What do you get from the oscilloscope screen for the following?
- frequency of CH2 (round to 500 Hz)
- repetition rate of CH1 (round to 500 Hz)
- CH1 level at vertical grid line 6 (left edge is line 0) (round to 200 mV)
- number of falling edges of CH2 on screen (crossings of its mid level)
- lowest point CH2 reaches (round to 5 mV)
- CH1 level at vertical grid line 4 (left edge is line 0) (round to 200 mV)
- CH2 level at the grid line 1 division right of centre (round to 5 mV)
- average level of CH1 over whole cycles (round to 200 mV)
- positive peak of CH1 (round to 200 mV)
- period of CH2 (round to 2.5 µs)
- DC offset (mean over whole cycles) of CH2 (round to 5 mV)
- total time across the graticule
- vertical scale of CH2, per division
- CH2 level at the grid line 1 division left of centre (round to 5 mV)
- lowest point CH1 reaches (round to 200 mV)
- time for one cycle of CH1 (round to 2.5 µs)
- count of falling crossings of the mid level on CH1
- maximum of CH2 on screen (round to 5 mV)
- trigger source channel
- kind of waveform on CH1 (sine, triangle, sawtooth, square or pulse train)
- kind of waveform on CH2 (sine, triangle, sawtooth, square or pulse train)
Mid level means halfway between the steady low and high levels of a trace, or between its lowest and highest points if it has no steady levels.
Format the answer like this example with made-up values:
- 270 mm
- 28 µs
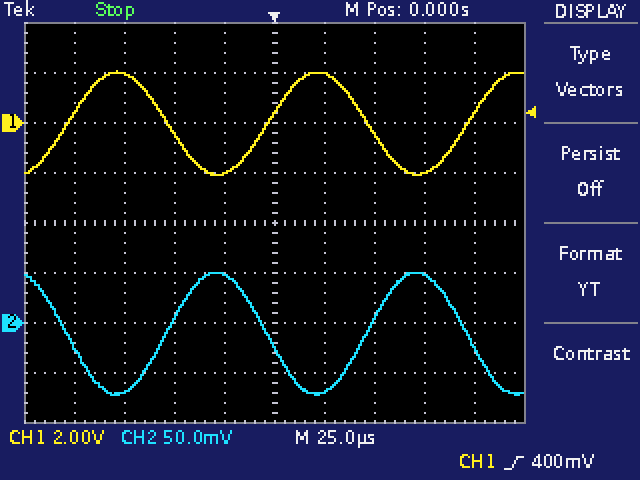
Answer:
- 10.0 kHz
- 10.0 kHz
- 2.0 V
- 3
- -70 mV
- -2.0 V
- -70 mV
- 0.0 V
- 2.0 V
- 100.0 µs
- -10 mV
- 250 µs
- 50 mV
- 50 mV
- -2.0 V
- 100.0 µs
- 2
- 50 mV
- CH1
- sine
- sine
